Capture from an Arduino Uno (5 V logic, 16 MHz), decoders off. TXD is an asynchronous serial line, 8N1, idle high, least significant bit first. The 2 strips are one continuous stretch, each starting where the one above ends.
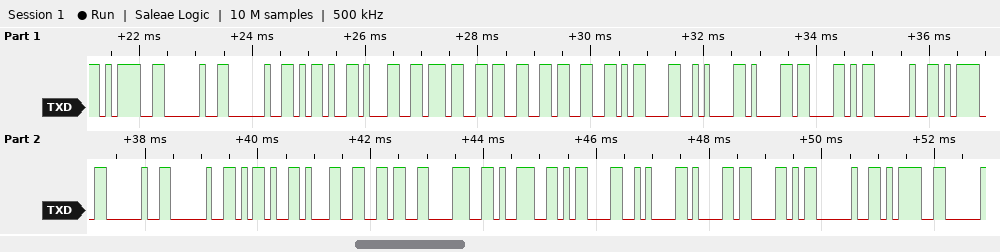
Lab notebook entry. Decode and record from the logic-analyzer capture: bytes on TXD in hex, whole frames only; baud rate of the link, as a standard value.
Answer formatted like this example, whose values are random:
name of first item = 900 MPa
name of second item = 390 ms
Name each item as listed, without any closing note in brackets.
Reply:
bytes on TXD in hex, whole frames only = 3D 20 20 2D 31 37 33 33 0D 0A 61 58 20 3D 20 20 2D 31 36 38 39 0D 0A 61 58 20 3D
baud rate of the link, as a standard value = 9600 baud
